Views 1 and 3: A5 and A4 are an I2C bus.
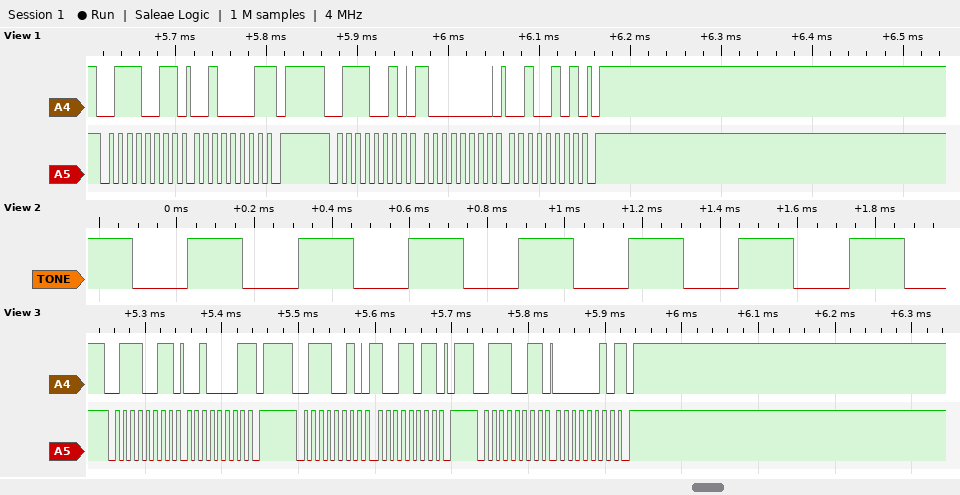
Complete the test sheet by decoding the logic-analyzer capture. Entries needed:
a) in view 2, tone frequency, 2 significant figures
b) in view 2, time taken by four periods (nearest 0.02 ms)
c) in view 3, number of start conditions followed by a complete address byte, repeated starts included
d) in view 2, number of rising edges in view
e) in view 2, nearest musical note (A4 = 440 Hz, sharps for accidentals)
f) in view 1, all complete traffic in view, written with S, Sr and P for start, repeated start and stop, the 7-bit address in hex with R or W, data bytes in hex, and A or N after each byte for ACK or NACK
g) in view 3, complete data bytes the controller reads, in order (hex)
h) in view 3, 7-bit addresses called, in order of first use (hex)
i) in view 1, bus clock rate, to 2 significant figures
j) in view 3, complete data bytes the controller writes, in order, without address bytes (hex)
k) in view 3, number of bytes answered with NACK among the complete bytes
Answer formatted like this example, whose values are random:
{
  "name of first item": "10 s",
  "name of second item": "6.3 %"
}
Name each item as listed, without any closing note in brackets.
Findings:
{
  "in view 2, tone frequency, 2 significant figures": "3.5 kHz",
  "in view 2, time taken by four periods": "1.14 ms",
  "in view 3, number of start conditions followed by a complete address byte, repeated starts included": "3",
  "in view 2, number of rising edges in view": "7",
  "in view 2, nearest musical note": "A7",
  "in view 1, all complete traffic in view, written with S, Sr and P for start, repeated start and stop, the 7-bit address in hex with R or W, data bytes in hex, and A or N after each byte for ACK or NACK": "S 39R A 21 N P S 39W A 80 A 25 A P",
  "in view 3, complete data bytes the controller reads, in order": "21 02",
  "in view 3, 7-bit addresses called, in order of first use": "0x39",
  "in view 1, bus clock rate, to 2 significant figures": "100 kHz",
  "in view 3, complete data bytes the controller writes, in order, without address bytes": "9B",
  "in view 3, number of bytes answered with NACK among the complete bytes": "2"
}
